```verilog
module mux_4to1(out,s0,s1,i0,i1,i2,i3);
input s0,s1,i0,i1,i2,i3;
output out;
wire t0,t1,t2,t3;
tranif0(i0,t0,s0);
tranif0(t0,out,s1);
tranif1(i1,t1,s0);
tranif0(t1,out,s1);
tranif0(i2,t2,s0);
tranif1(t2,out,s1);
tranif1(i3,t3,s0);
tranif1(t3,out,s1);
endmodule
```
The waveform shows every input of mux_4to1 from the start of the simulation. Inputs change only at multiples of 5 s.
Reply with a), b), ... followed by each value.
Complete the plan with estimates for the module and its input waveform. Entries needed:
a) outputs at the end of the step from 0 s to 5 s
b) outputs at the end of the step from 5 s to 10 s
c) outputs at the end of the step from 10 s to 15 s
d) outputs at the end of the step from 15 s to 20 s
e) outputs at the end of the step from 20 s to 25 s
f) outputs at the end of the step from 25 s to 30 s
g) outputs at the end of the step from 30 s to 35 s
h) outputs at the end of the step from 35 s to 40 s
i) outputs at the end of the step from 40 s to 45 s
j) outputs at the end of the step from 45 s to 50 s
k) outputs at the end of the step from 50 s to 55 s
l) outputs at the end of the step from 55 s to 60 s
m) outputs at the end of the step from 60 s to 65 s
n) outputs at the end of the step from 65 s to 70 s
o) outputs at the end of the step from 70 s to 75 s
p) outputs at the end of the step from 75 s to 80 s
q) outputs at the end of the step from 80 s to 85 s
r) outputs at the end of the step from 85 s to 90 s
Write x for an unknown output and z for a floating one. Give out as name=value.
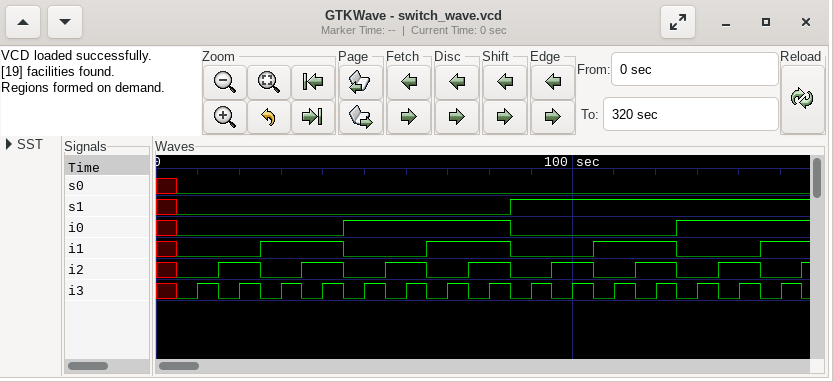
a) out=x
b) out=0
c) out=0
d) out=0
e) out=0
f) out=0
g) out=0
h) out=0
i) out=0
j) out=1
k) out=1
l) out=1
m) out=1
n) out=1
o) out=1
p) out=1
q) out=1
r) out=0
